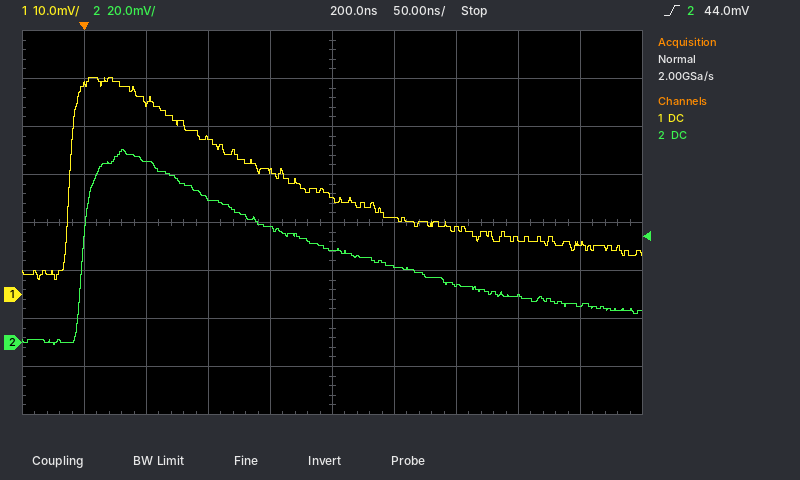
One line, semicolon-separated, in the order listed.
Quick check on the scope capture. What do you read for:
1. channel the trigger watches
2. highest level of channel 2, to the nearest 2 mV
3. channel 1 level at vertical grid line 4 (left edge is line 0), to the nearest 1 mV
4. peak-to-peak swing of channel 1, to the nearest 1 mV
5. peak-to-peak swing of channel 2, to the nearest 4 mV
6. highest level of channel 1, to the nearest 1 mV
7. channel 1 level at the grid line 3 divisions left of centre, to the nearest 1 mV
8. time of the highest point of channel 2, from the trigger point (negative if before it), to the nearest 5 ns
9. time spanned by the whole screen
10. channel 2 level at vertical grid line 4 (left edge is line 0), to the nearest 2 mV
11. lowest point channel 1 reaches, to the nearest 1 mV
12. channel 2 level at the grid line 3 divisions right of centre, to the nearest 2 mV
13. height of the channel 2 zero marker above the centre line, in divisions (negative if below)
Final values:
channel 2; 80 mV; 26 mV; 42 mV; 80 mV; 45 mV; 40 mV; +30 ns; 500 ns; 48 mV; 3 mV; 20 mV; -2.5 div
